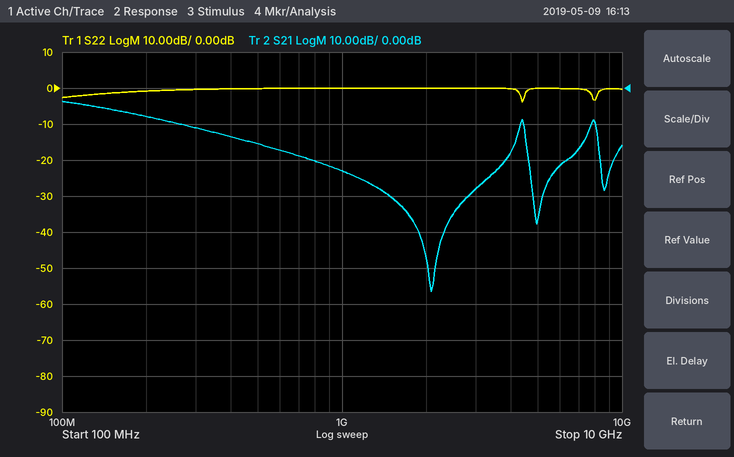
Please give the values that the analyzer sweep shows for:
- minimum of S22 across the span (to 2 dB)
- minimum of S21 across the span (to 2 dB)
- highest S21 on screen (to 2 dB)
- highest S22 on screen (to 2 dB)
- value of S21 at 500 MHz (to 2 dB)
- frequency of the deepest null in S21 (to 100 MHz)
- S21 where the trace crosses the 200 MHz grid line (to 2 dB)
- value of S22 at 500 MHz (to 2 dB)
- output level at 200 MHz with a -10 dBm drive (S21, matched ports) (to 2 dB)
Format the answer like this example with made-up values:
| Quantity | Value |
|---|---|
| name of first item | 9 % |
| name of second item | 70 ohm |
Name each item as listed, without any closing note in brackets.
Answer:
| Quantity | Value |
|---|---|
| minimum of S22 across the span | -4 dB |
| minimum of S21 across the span | -56 dB |
| highest S21 on screen | -4 dB |
| highest S22 on screen | 0 dB |
| value of S21 at 500 MHz | -16 dB |
| frequency of the deepest null in S21 | 2.1 GHz |
| S21 where the trace crosses the 200 MHz grid line | -8 dB |
| value of S22 at 500 MHz | 0 dB |
| output level at 200 MHz with a -10 dBm drive (S21, matched ports) | -18 dBm |
